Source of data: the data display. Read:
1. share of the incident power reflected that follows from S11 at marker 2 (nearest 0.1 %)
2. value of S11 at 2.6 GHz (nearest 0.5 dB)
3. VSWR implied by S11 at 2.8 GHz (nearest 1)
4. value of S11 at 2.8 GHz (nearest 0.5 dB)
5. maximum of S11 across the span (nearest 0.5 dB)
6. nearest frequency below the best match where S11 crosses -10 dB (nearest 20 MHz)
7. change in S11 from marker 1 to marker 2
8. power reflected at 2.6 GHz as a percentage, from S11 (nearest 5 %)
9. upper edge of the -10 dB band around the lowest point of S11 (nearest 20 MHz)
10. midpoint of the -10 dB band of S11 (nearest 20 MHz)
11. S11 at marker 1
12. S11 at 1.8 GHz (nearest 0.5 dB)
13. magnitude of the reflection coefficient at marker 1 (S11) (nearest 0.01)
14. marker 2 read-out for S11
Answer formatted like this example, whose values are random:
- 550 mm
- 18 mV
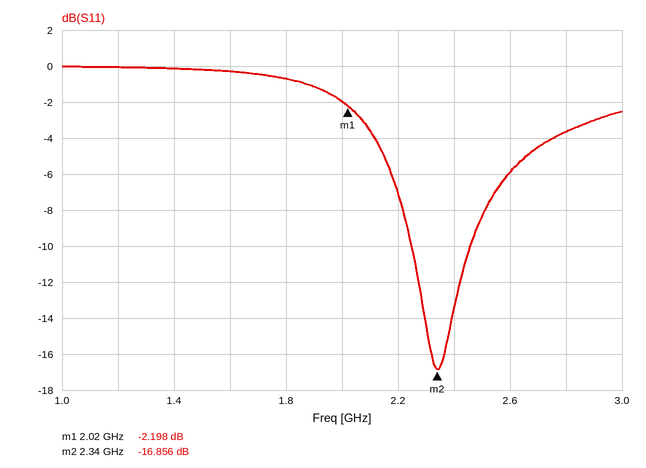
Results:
- 2.1 %
- -6.0 dB
- 5
- -3.5 dB
- 0.0 dB
- 2.24 GHz
- -14.658 dB
- 25 %
- 2.46 GHz
- 2.36 GHz
- -2.198 dB
- -0.5 dB
- 0.78
- -16.856 dB
